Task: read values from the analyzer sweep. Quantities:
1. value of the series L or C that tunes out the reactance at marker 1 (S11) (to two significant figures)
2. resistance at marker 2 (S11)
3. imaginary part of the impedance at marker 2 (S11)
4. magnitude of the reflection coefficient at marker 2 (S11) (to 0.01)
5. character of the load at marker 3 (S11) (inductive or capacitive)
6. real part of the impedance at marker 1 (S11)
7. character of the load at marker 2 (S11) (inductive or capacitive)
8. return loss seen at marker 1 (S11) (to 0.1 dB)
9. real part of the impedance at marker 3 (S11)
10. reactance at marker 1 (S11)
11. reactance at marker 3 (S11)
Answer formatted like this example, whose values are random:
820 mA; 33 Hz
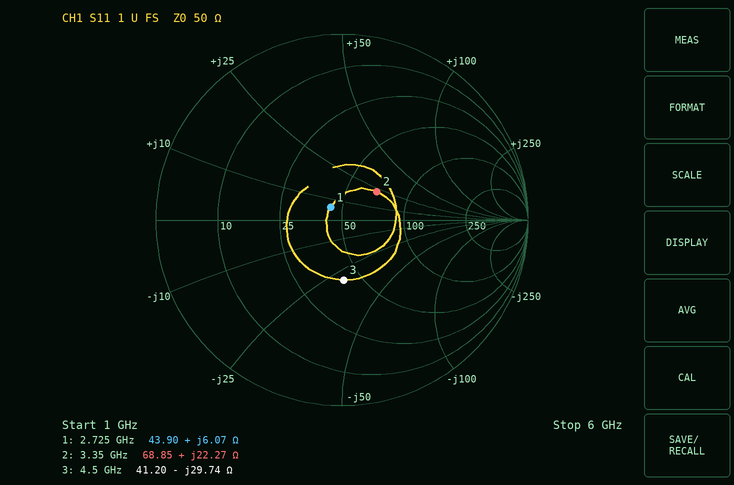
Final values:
9.6 pF; 68.85 Ω; +22.27 Ω; 0.24; capacitive; 43.90 Ω; inductive; 20.8 dB; 41.20 Ω; +6.07 Ω; -29.74 Ω
